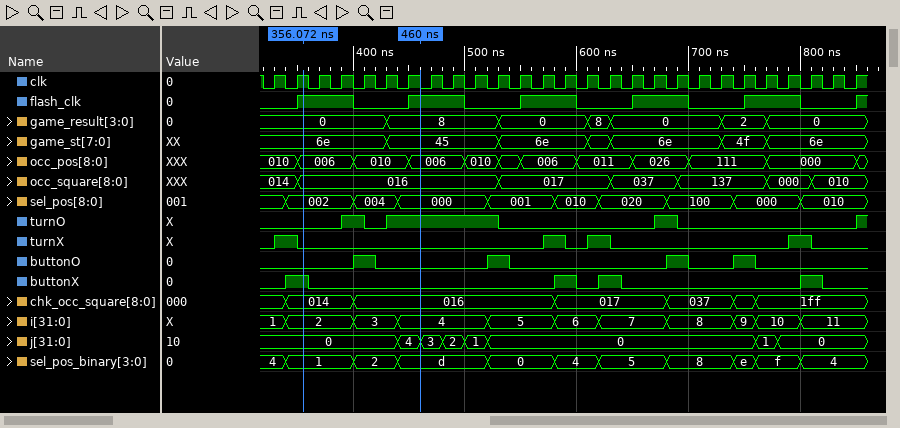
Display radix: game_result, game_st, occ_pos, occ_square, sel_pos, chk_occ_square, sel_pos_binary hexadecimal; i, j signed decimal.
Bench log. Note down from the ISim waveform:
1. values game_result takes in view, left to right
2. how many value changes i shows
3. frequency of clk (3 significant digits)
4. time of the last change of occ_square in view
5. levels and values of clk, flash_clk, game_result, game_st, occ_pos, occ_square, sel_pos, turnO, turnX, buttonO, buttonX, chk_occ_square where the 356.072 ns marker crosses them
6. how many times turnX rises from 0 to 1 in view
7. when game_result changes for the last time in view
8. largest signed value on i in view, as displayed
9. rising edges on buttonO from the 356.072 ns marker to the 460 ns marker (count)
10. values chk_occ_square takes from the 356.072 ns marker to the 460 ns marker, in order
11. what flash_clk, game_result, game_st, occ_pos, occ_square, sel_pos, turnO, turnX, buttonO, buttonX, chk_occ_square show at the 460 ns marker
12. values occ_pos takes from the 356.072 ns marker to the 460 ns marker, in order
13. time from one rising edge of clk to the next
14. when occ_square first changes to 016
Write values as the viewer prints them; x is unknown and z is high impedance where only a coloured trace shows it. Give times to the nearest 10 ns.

0, 8, 0, 8, 0, 2, 0
10
50.0 MHz
810 ns
clk=1, flash_clk=1, game_result=0, game_st=6e, occ_pos=006, occ_square=016, sel_pos=002, turnO=0, turnX=0, buttonO=0, buttonX=1, chk_occ_square=014
4
770 ns
11
1
014, 016
flash_clk=1, game_result=8, game_st=45, occ_pos=006, occ_square=016, sel_pos=000, turnO=1, turnX=0, buttonO=0, buttonX=0, chk_occ_square=016
006, 010, 006
20 ns
350 ns
